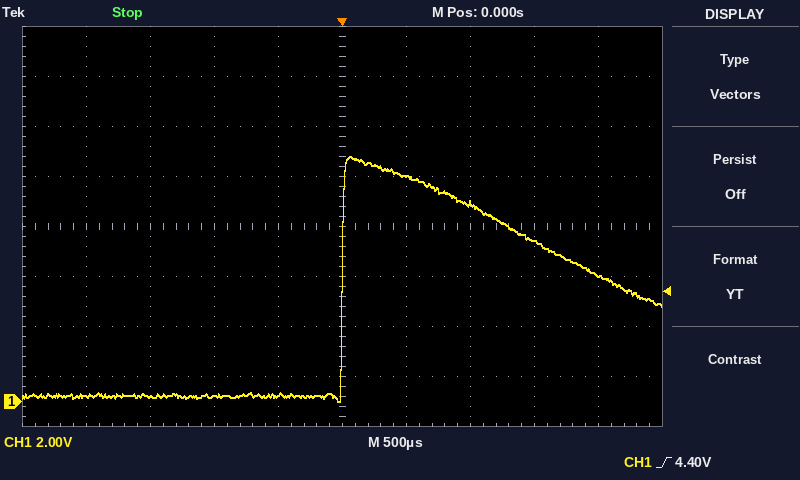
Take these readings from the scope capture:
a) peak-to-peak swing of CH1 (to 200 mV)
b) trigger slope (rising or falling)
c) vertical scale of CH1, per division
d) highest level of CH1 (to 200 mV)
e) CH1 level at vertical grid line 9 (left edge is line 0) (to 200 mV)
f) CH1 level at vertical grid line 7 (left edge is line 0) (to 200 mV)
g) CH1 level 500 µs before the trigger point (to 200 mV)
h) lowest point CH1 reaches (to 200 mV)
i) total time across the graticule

9.8 V
rising
2 V
9.8 V
5.0 V
8.0 V
200 mV
0.0 V
5 ms
